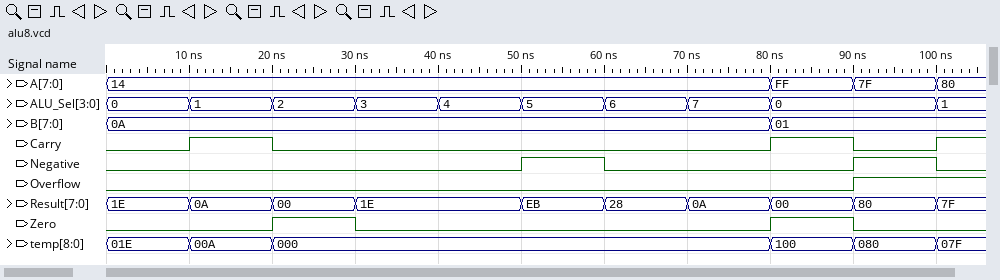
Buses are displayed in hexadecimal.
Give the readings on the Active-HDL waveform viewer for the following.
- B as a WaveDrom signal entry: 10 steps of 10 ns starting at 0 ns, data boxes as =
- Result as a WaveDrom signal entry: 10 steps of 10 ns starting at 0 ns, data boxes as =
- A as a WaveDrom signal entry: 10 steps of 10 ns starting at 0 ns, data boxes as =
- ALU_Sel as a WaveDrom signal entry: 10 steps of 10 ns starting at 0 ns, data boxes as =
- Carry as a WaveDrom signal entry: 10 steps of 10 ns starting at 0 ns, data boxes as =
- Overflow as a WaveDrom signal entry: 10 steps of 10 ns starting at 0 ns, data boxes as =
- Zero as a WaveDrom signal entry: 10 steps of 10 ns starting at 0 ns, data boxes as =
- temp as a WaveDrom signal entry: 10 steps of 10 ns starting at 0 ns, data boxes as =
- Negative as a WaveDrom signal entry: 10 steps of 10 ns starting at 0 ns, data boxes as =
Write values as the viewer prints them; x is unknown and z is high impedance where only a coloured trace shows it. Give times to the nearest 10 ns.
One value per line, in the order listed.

{name: 'B', wave: '=.......=.', data: '0A 01'}
{name: 'Result', wave: '====.=====', data: '1E 0A 00 1E EB 28 0A 00 80'}
{name: 'A', wave: '=.......==', data: '14 FF 7F'}
{name: 'ALU_Sel', wave: '=========.', data: '0 1 2 3 4 5 6 7 0'}
{name: 'Carry', wave: '010.....10'}
{name: 'Overflow', wave: '0........1'}
{name: 'Zero', wave: '0.10....10'}
{name: 'temp', wave: '===.....==', data: '01E 00A 000 100 080'}
{name: 'Negative', wave: '0....10..1'}
